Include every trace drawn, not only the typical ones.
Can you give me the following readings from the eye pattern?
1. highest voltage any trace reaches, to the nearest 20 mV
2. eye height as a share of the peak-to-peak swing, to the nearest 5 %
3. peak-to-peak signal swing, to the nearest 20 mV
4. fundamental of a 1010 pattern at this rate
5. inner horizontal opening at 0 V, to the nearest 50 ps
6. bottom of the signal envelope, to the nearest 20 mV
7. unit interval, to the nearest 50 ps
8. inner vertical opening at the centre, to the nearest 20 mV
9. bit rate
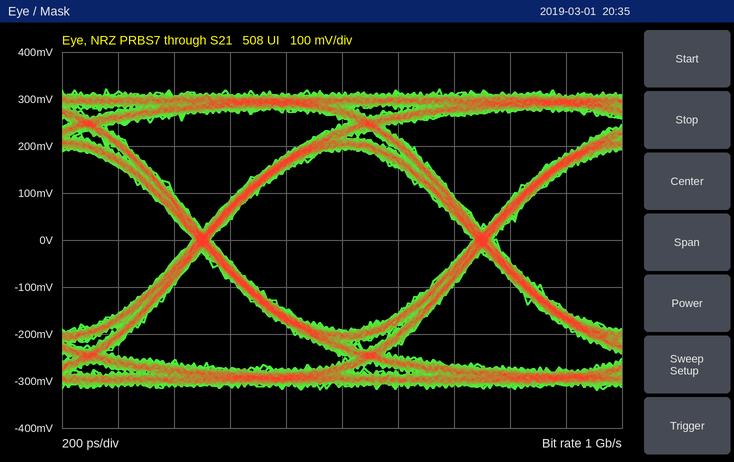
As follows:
320 mV
60 %
640 mV
500 MHz
950 ps
-320 mV
1.00 ns
380 mV
1 Gb/s
